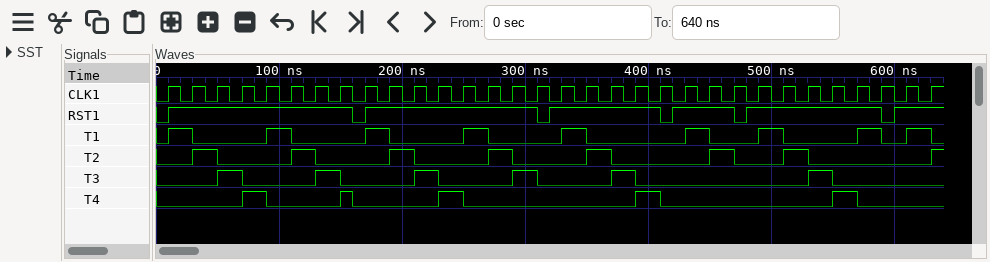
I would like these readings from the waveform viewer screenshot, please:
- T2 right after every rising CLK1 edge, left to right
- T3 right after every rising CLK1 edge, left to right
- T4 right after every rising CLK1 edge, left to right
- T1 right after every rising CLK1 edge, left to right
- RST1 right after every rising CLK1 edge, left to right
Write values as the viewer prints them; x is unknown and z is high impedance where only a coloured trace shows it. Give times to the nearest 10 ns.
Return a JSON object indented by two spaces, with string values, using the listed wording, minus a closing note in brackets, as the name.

{
  "T2 right after every rising CLK1 edge, left to right": "0 1 0 0 0 1 0 0 0 1 0 0 0 1 0 0 0 1 0 0 0 0 1 0 0 1 0 0 0 0 0 1",
  "T3 right after every rising CLK1 edge, left to right": "0 0 1 0 0 0 1 0 0 0 1 0 0 0 1 0 0 0 1 0 0 0 0 0 0 0 1 0 0 0 0 0",
  "T4 right after every rising CLK1 edge, left to right": "0 0 0 1 0 0 0 1 0 0 0 1 0 0 0 0 0 0 0 1 0 0 0 0 0 0 0 1 0 0 0 0",
  "T1 right after every rising CLK1 edge, left to right": "1 0 0 0 1 0 0 0 1 0 0 0 1 0 0 0 1 0 0 0 0 1 0 0 1 0 0 0 1 0 1 0",
  "RST1 right after every rising CLK1 edge, left to right": "1 1 1 1 1 1 1 1 1 1 1 1 1 1 1 0 1 1 1 1 0 1 1 0 1 1 1 1 1 0 1 1"
}
